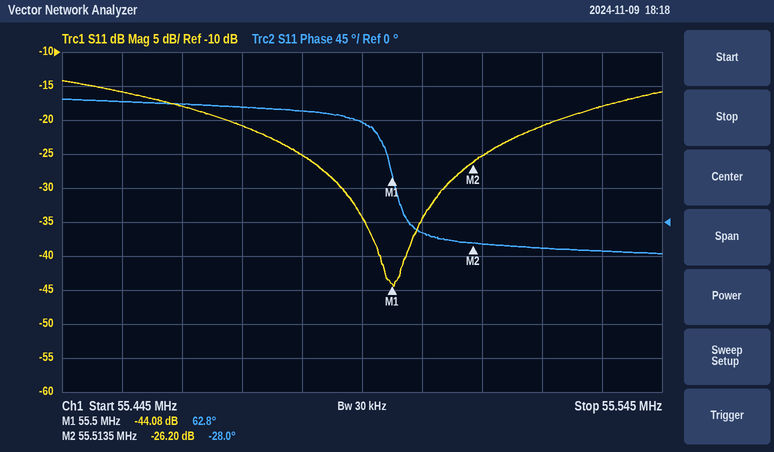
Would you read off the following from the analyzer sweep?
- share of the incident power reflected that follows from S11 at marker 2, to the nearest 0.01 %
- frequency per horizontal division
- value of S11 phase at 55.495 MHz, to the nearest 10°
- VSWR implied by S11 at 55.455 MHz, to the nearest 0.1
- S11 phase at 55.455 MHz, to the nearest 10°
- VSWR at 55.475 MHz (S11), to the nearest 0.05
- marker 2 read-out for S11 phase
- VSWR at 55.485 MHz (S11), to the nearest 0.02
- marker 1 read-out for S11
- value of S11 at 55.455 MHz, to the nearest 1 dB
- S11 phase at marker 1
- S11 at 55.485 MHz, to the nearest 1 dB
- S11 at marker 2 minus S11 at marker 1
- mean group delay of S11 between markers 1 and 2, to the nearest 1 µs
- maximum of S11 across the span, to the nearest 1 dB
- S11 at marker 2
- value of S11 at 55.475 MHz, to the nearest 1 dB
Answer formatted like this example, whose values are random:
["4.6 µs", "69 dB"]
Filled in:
["0.24 %", "10 kHz", "130°", "1.4", "160°", "1.20", "-28.0°", "1.12", "-44.08 dB", "-16 dB", "62.8°", "-25 dB", "17.88 dB", "19 µs", "-14 dB", "-26.20 dB", "-21 dB"]
